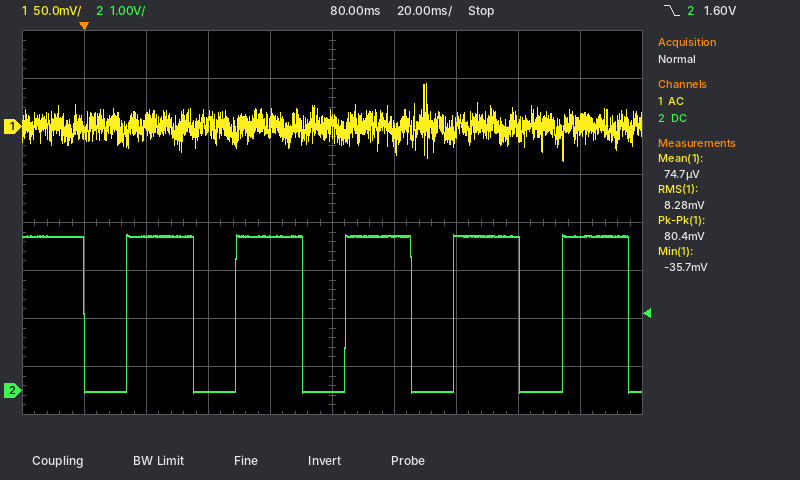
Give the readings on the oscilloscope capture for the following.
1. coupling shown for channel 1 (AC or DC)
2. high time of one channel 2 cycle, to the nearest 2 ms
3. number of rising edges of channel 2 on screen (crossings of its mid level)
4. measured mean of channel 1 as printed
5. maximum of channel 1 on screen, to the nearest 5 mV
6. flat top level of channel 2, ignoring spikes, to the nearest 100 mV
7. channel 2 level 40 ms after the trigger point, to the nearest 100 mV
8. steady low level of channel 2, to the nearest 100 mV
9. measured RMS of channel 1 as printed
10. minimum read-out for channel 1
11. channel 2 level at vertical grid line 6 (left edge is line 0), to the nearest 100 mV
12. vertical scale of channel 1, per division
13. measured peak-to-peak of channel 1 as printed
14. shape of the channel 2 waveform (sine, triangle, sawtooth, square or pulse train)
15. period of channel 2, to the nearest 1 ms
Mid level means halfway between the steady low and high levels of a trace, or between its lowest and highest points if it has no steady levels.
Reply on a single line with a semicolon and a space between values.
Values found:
AC; 22 ms; 5; 74.7 µV; 45 mV; 3.2 V; 0.0 V; 0.0 V; 8.28 mV; -35.7 mV; 3.2 V; 50 mV; 80.4 mV; pulse train; 35 ms
